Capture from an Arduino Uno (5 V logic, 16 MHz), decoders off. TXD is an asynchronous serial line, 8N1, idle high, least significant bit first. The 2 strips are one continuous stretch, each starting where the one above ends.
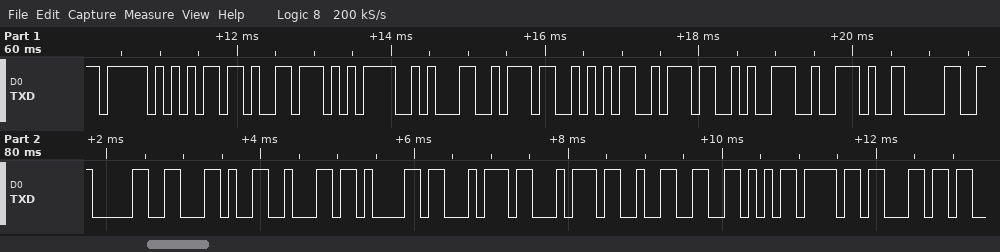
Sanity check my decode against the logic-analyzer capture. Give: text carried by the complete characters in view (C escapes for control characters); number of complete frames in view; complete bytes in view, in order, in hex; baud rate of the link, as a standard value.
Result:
"_mv=17579.00,batt2Vol"
21
0x5F 0x6D 0x76 0x3D 0x31 0x37 0x35 0x37 0x39 0x2E 0x30 0x30 0x2C 0x62 0x61 0x74 0x74 0x32 0x56 0x6F 0x6C
9600 baud
